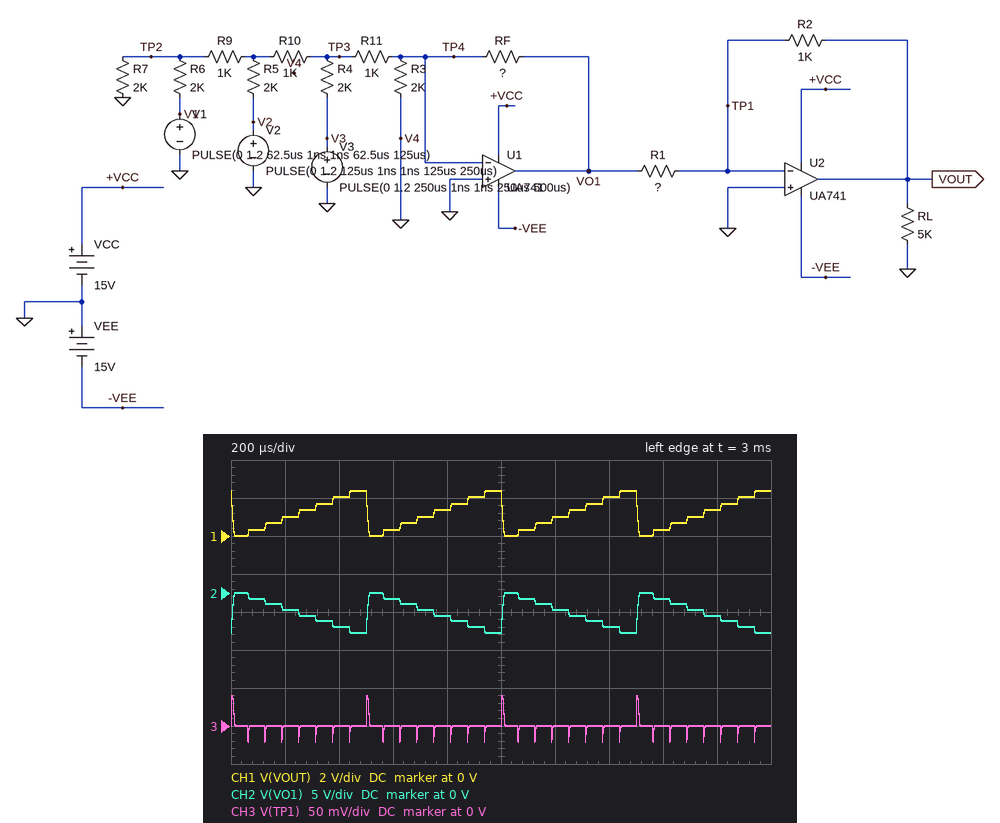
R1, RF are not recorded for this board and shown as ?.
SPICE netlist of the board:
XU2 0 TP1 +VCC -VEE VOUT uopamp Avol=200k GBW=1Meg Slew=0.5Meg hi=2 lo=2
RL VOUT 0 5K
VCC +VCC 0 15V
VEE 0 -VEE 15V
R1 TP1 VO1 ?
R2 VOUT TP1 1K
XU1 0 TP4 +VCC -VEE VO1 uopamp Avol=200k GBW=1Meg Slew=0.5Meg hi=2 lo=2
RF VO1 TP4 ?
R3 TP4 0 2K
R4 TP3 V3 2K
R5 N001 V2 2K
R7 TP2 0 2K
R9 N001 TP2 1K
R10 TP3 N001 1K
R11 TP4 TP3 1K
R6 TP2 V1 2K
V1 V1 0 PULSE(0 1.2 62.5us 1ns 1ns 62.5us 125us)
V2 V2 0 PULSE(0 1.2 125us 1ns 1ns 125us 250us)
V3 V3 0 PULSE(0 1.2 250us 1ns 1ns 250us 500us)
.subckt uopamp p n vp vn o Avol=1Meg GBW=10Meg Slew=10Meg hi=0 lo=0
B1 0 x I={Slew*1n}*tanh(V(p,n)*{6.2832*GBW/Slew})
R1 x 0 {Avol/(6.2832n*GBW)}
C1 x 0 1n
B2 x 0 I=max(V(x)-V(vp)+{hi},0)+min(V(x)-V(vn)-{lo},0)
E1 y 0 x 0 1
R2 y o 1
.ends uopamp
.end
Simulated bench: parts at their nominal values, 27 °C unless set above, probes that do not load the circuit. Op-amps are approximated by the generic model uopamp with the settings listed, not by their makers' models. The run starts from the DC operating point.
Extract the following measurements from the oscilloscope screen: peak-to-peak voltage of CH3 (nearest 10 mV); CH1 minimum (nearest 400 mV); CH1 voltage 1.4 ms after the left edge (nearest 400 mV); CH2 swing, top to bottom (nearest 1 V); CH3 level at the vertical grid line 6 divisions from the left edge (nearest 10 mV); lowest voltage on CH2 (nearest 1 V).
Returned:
60 mV
0 V
2.0 V
5 V
0 V
-5 V
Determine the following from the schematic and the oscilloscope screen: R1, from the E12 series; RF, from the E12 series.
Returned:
2.2 kΩ
10 kΩ
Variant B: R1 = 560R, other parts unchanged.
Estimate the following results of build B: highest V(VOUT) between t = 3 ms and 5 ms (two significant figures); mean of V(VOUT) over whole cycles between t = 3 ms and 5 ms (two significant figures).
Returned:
9.4 V
4.8 V
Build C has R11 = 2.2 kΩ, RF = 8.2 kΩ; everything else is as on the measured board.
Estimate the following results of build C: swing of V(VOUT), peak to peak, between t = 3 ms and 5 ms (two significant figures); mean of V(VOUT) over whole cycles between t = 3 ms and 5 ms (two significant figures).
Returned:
1.2 V
620 mV
